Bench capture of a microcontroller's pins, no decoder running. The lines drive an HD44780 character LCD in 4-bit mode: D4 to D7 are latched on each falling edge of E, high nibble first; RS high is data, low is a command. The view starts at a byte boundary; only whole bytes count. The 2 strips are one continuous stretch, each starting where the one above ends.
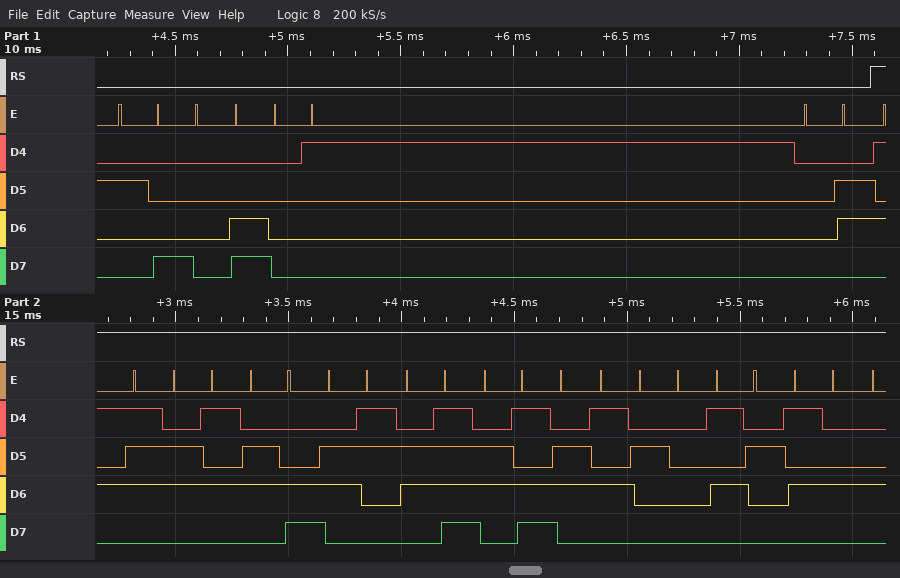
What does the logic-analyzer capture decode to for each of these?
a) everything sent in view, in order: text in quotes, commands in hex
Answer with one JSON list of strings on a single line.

["0x28 0x0C 0x01 0x06 \"Welcome RT\""]
